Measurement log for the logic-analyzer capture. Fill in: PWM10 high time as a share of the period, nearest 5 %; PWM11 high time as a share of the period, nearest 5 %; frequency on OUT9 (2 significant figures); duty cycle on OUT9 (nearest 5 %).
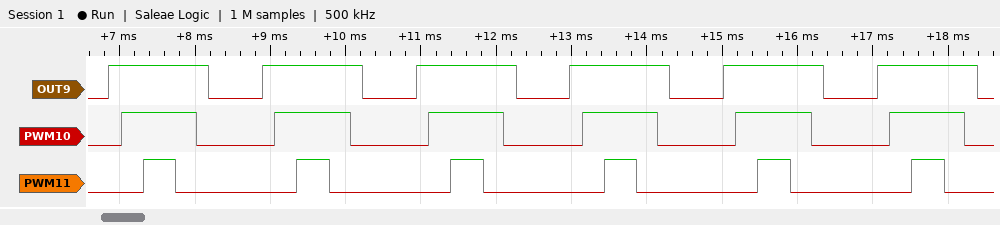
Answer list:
50 %
20 %
490 Hz
65 %
